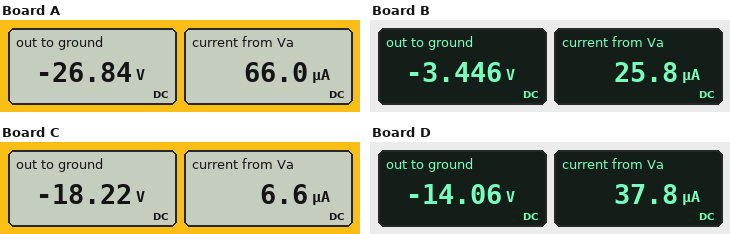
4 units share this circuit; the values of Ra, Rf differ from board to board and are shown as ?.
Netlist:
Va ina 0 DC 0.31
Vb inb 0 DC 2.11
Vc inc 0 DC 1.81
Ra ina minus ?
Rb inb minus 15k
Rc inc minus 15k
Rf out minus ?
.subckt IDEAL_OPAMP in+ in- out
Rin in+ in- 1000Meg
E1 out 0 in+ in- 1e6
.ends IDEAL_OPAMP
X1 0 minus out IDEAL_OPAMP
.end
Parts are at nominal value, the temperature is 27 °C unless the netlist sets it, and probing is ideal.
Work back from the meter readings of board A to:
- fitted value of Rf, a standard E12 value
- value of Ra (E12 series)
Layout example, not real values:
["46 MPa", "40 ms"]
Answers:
["82 kΩ", "4.7 kΩ"]
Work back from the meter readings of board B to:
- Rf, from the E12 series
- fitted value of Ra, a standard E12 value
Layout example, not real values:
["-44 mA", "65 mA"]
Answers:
["12 kΩ", "12 kΩ"]
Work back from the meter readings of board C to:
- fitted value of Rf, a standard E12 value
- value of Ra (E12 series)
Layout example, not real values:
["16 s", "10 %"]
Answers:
["68 kΩ", "47 kΩ"]
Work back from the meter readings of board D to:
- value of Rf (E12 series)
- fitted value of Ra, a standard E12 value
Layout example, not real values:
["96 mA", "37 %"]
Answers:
["47 kΩ", "8.2 kΩ"]
